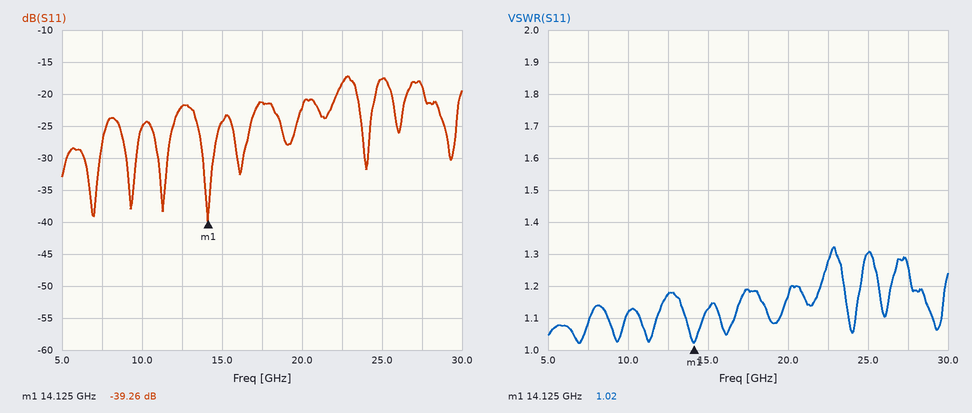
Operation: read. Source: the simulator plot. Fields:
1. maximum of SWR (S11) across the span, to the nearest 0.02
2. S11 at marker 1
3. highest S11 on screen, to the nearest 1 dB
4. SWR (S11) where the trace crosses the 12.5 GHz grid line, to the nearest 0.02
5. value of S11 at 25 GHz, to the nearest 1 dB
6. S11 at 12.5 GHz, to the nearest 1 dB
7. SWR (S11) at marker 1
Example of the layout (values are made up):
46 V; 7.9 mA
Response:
1.32; -39.26 dB; -17 dB; 1.18; -18 dB; -22 dB; 1.02
